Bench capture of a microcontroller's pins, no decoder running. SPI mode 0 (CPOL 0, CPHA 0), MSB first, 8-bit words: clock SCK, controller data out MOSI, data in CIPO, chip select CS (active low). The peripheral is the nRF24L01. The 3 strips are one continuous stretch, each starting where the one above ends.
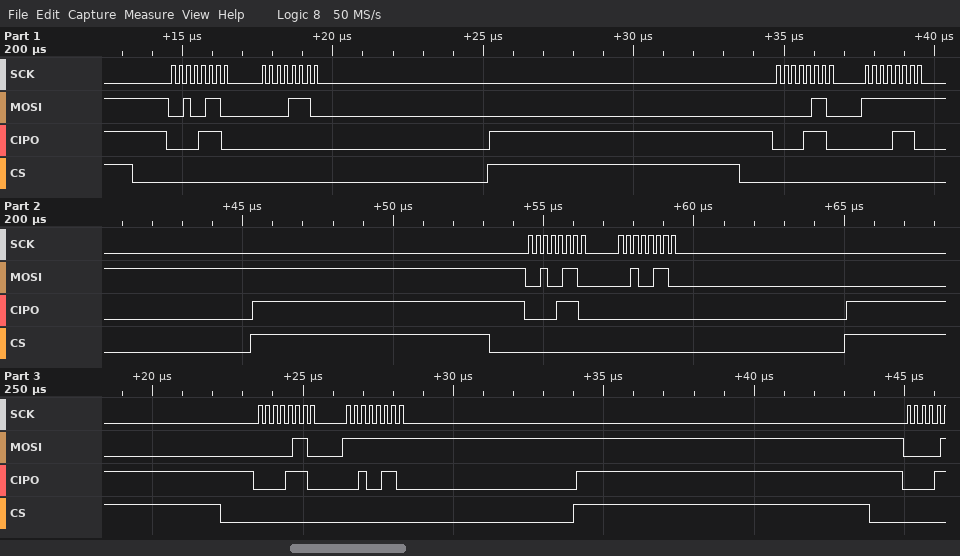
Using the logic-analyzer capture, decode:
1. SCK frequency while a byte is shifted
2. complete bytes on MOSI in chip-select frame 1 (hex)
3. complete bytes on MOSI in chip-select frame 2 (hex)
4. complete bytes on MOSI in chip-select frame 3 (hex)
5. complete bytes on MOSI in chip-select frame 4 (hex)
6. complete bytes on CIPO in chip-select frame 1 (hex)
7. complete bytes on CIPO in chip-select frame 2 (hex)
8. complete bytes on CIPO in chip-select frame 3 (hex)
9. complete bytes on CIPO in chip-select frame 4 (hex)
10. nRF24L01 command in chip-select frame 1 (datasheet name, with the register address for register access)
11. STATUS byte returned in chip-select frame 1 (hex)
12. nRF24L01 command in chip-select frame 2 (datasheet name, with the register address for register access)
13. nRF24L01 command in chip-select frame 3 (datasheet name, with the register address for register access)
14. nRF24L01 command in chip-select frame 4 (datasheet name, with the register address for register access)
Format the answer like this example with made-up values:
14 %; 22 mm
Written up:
4 MHz; 26 0E; 06 FF; 26 26; 06 FF; 0E 00; 0E 0E; 0E 00; 0E 26; W_REGISTER 0x06; 0x0E; R_REGISTER 0x06; W_REGISTER 0x06; R_REGISTER 0x06
